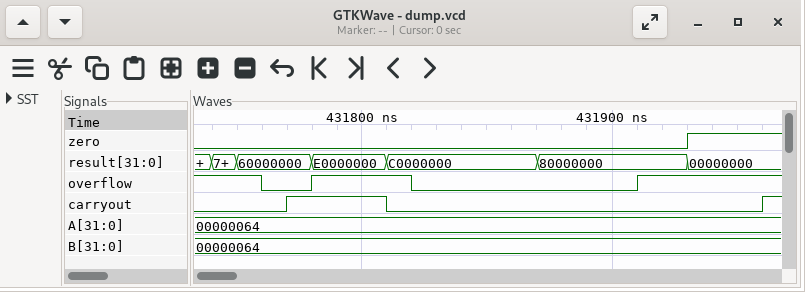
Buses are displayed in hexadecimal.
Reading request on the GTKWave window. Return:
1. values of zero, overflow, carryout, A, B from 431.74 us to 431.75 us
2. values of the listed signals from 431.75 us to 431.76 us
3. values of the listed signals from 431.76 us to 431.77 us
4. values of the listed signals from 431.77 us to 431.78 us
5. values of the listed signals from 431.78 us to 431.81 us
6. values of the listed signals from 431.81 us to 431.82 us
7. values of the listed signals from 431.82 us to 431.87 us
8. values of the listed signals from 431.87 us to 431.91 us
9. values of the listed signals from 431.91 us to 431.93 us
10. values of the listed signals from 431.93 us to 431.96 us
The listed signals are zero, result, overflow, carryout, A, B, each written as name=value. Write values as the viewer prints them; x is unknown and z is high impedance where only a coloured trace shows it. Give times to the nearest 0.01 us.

zero=0, overflow=1, carryout=0, A=00000064, B=00000064
zero=0, result=60000000, overflow=1, carryout=0, A=00000064, B=00000064
zero=0, result=60000000, overflow=0, carryout=0, A=00000064, B=00000064
zero=0, result=60000000, overflow=0, carryout=1, A=00000064, B=00000064
zero=0, result=E0000000, overflow=1, carryout=1, A=00000064, B=00000064
zero=0, result=C0000000, overflow=1, carryout=0, A=00000064, B=00000064
zero=0, result=C0000000, overflow=0, carryout=0, A=00000064, B=00000064
zero=0, result=80000000, overflow=0, carryout=0, A=00000064, B=00000064
zero=0, result=80000000, overflow=1, carryout=0, A=00000064, B=00000064
zero=1, result=00000000, overflow=1, carryout=0, A=00000064, B=00000064
